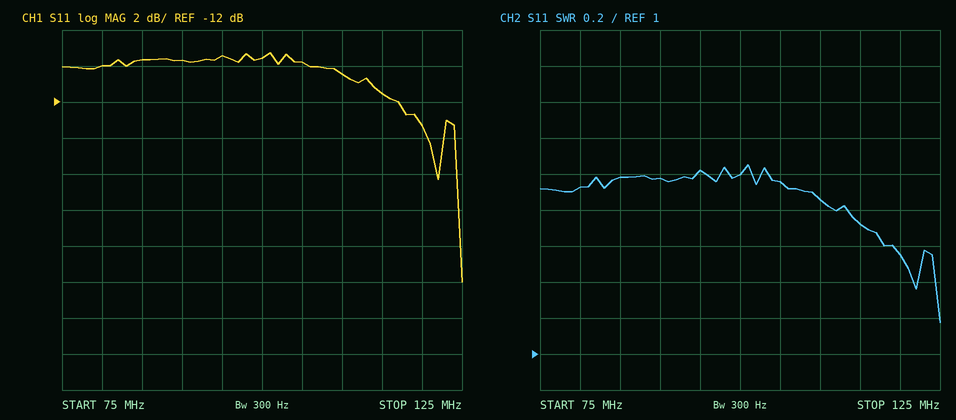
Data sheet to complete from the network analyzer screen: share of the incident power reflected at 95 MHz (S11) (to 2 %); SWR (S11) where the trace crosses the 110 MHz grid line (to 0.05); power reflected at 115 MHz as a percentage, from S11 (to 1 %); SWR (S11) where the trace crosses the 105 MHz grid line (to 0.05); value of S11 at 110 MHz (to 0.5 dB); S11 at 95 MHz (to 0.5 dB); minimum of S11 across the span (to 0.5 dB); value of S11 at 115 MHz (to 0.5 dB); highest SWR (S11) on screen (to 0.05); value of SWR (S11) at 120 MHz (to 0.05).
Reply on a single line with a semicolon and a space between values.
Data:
12 %; 1.85; 7 %; 1.95; -10.5 dB; -9.5 dB; -22.0 dB; -11.5 dB; 2.05; 1.55
